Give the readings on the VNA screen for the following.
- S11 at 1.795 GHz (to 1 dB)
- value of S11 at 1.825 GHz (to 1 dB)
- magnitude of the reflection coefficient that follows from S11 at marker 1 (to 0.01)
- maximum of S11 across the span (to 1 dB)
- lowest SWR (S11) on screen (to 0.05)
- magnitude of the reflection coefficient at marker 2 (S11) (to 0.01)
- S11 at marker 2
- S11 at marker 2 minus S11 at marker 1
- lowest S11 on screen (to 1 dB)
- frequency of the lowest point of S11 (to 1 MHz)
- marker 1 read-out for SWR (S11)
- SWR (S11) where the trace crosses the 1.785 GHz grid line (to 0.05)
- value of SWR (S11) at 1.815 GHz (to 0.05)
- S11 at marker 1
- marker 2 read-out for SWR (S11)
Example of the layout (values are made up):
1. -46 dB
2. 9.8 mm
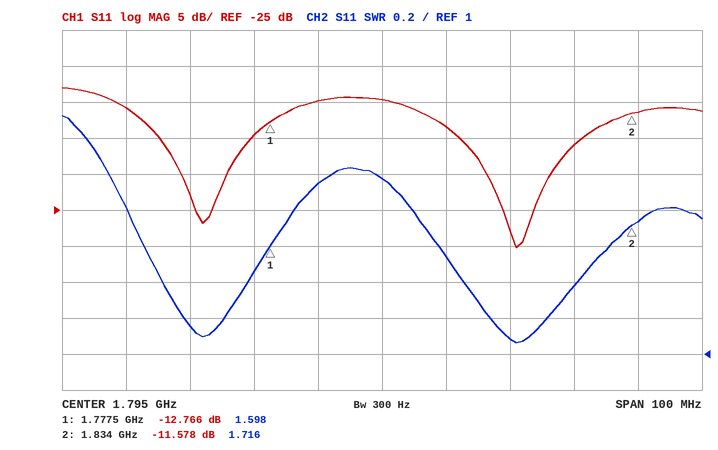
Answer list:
1. -10 dB
2. -16 dB
3. 0.23
4. -8 dB
5. 1.05
6. 0.26
7. -11.578 dB
8. 1.188 dB
9. -30 dB
10. 1.816 GHz
11. 1.598
12. 1.95
13. 1.10
14. -12.766 dB
15. 1.716
